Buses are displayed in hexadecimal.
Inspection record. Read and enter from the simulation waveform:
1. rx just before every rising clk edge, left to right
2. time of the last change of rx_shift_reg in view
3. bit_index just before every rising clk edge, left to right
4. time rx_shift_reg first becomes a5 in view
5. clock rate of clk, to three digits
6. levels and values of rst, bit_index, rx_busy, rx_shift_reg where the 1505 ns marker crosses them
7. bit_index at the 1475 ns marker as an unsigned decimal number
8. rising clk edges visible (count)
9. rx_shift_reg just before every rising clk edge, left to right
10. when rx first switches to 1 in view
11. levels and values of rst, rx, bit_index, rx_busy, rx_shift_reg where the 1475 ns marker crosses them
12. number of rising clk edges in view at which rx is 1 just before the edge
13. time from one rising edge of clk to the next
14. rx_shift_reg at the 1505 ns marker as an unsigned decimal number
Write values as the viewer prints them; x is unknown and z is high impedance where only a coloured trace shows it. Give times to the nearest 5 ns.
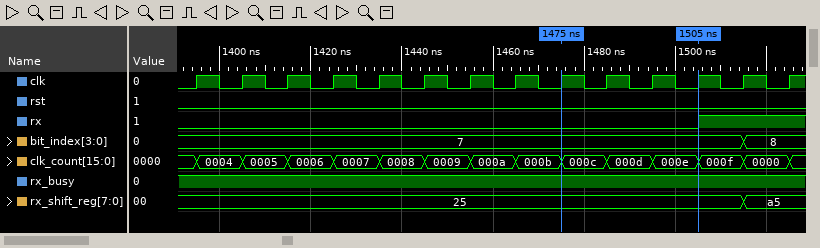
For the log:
0 0 0 0 0 0 0 0 0 0 0 0 1 1
1515 ns
7, 7, 7, 7, 7, 7, 7, 7, 7, 7, 7, 7, 7, 8
1515 ns
100 MHz
rst=0, bit_index=7, rx_busy=1, rx_shift_reg=25
7
14
25, 25, 25, 25, 25, 25, 25, 25, 25, 25, 25, 25, 25, a5
1505 ns
rst=0, rx=0, bit_index=7, rx_busy=1, rx_shift_reg=25
2
10 ns
37
